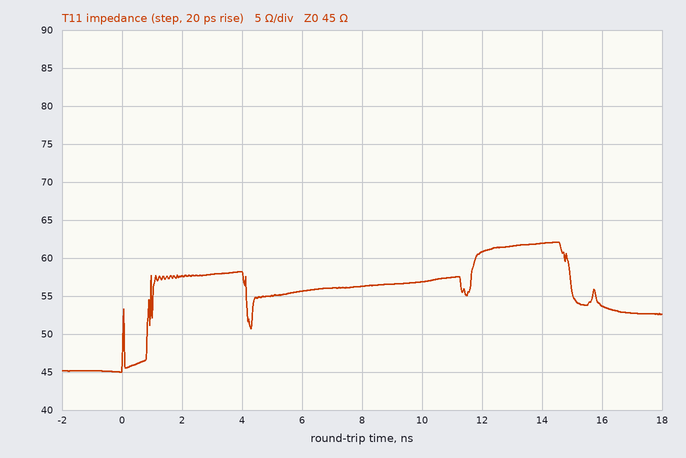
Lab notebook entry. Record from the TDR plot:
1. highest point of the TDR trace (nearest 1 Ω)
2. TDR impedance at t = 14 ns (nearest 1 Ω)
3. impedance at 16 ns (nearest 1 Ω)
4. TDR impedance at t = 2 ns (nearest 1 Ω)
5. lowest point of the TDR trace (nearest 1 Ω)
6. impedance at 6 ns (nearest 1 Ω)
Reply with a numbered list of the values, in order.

1. 62 Ω
2. 62 Ω
3. 54 Ω
4. 58 Ω
5. 45 Ω
6. 56 Ω
